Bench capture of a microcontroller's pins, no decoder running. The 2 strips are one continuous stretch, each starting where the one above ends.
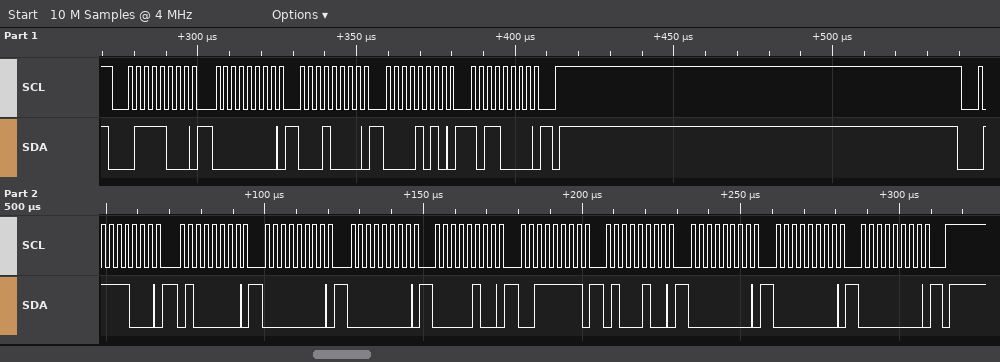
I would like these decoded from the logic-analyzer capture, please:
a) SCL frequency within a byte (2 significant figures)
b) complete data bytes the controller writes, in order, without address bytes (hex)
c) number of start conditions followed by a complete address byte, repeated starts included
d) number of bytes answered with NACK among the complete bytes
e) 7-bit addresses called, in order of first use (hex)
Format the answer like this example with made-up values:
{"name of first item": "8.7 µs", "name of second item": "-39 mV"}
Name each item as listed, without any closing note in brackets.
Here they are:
{"SCL frequency within a byte": "400 kHz", "complete data bytes the controller writes, in order, without address bytes": "00 10 0A B0 40 00 00 04 3F 44 00 00 00", "number of start conditions followed by a complete address byte, repeated starts included": "2", "number of bytes answered with NACK among the complete bytes": "0", "7-bit addresses called, in order of first use": "0x3C"}
